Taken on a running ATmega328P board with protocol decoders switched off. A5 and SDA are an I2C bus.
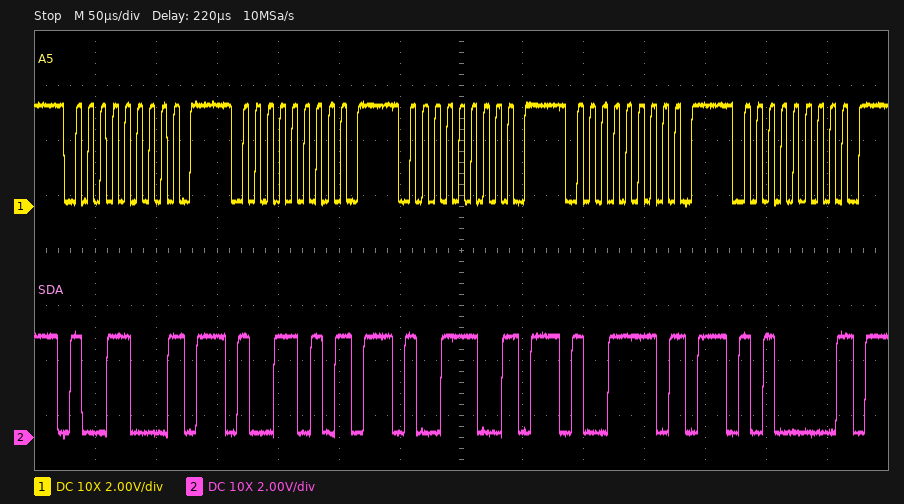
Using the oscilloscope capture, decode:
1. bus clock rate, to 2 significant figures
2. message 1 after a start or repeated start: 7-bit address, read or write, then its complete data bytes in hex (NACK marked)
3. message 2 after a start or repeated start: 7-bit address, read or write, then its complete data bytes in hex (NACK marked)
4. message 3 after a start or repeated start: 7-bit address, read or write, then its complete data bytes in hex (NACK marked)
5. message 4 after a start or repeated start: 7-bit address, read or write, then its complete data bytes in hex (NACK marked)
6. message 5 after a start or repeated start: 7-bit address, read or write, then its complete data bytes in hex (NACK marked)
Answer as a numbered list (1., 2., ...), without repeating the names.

1. 100 kHz
2. 0x4C write NACK
3. 0x4D write NACK
4. 0x4E write NACK
5. 0x4F write NACK
6. 0x50 write NACK
